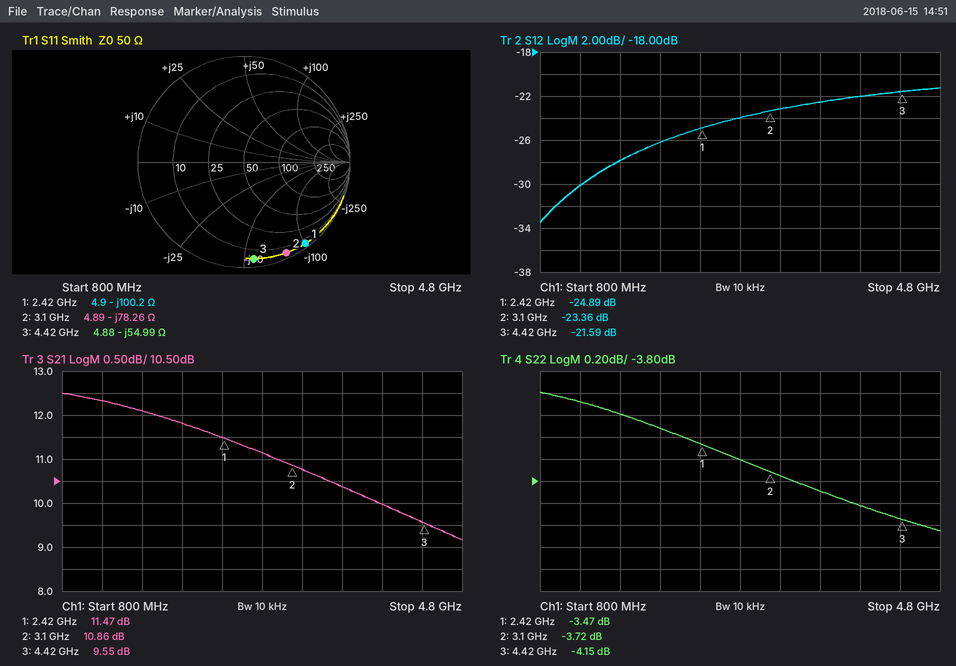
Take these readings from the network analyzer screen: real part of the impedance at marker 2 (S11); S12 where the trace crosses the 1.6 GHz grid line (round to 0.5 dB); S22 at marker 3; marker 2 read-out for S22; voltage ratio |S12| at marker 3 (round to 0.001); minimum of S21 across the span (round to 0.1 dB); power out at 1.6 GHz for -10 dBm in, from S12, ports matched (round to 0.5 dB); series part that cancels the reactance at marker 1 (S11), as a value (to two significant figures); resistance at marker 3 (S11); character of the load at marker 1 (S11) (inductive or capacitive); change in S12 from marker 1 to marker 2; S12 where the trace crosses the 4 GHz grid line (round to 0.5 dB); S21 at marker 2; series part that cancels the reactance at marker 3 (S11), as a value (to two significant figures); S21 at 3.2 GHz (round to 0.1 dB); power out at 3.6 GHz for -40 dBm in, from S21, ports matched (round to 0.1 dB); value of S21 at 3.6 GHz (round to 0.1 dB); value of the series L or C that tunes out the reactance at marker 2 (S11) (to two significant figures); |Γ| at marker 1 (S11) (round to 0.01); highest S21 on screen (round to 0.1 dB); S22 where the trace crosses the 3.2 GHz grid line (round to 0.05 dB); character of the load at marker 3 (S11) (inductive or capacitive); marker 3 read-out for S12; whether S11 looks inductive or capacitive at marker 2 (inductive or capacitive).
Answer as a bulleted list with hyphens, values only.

- 4.89 Ω
- -28.0 dB
- -4.15 dB
- -3.72 dB
- 0.083
- 9.2 dB
- -38.0 dBm
- 6.6 nH
- 4.88 Ω
- capacitive
- 1.53 dB
- -22.0 dB
- 10.86 dB
- 2.0 nH
- 10.8 dB
- -29.6 dBm
- 10.4 dB
- 4.0 nH
- 0.96
- 12.5 dB
- -3.75 dB
- capacitive
- -21.59 dB
- capacitive
